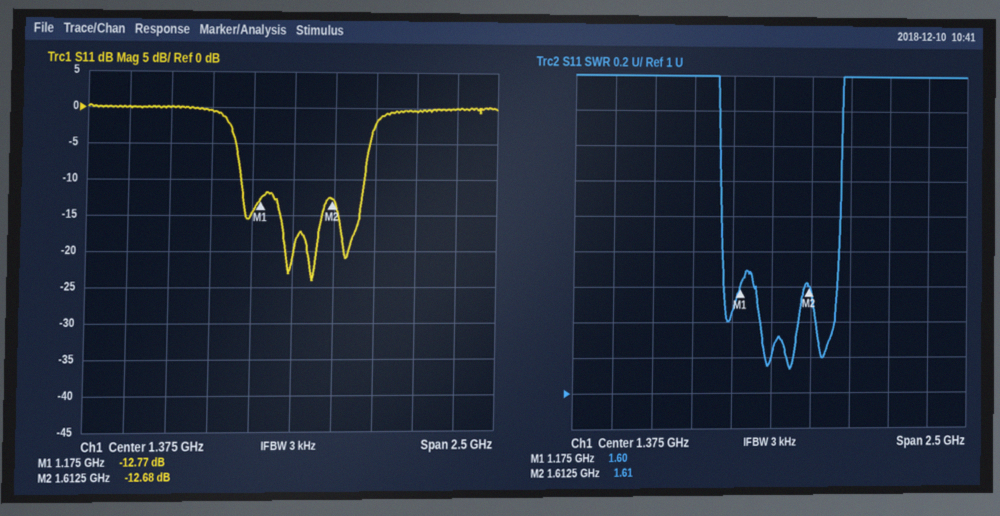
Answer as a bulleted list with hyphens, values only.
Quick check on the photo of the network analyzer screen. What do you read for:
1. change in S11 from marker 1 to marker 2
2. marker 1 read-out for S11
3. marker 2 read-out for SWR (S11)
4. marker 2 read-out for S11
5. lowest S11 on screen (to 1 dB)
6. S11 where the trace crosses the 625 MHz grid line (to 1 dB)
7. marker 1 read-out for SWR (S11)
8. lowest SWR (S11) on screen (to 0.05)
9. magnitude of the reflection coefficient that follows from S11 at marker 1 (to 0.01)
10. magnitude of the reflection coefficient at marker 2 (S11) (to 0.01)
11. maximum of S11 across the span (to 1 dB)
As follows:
- 0.09 dB
- -12.77 dB
- 1.61
- -12.68 dB
- -24 dB
- 0 dB
- 1.60
- 1.15
- 0.23
- 0.23
- 0 dB
